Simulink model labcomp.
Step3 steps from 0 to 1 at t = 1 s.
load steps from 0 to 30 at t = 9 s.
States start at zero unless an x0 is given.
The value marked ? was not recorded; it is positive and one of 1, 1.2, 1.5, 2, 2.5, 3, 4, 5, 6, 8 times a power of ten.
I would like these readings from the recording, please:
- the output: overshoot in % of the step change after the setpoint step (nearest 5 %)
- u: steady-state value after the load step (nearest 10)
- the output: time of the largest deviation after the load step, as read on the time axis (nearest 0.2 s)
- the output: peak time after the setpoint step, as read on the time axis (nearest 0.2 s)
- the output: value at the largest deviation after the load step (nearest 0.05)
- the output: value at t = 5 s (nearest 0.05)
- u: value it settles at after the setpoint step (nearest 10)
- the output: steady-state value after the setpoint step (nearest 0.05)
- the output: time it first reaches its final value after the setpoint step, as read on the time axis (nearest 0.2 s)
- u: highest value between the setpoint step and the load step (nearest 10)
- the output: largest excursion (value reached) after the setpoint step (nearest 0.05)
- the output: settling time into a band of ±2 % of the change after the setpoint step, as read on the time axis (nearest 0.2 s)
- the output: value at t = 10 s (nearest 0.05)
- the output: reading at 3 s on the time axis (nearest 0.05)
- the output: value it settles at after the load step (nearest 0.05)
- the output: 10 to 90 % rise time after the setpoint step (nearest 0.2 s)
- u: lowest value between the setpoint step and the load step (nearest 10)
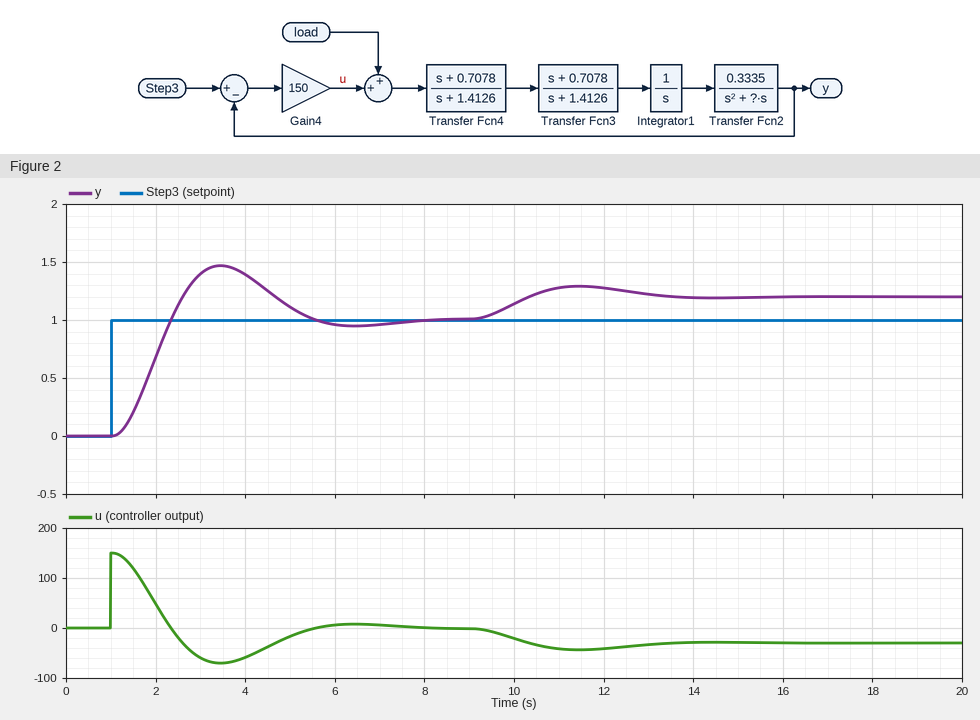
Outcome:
45 %
-30
11.4 s
3.4 s
1.30
1.10
0
1.00
2.4 s
150
1.45
7.6 s
1.15
1.40
1.20
0.8 s
-70
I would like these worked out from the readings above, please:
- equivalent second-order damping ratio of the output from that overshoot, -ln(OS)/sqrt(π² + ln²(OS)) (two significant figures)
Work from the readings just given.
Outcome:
0.25
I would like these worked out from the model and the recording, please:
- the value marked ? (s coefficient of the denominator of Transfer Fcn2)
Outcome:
20
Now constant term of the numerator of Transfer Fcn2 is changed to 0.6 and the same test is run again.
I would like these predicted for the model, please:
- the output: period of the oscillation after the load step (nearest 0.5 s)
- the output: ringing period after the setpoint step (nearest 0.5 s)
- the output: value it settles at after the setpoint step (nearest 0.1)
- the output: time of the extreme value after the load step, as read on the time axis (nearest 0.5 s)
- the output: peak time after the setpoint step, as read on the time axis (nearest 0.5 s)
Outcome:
3.5 s
3.5 s
1.0
10.5 s
2.5 s
